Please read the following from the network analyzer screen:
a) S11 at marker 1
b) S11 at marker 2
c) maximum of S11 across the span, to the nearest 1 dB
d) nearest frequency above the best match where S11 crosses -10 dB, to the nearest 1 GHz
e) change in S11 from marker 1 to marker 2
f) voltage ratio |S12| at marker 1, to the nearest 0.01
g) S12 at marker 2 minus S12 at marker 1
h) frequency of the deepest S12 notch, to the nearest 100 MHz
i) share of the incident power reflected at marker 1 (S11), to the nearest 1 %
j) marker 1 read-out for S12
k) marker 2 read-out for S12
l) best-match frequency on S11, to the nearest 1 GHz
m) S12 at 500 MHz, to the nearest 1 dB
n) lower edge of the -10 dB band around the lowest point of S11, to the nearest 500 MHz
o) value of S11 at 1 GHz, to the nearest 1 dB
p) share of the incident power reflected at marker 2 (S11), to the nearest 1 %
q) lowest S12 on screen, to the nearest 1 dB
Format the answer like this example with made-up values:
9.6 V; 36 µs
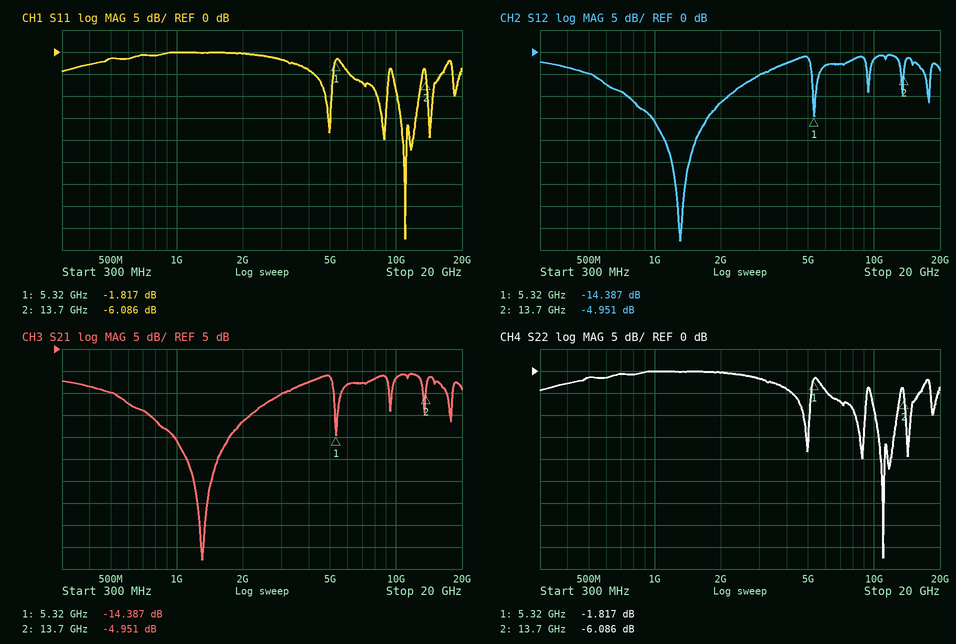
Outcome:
-1.817 dB; -6.086 dB; 0 dB; 13 GHz; -4.269 dB; 0.19; 9.436 dB; 1.3 GHz; 66 %; -14.387 dB; -4.951 dB; 11 GHz; -5 dB; 10.0 GHz; 0 dB; 25 %; -43 dB
